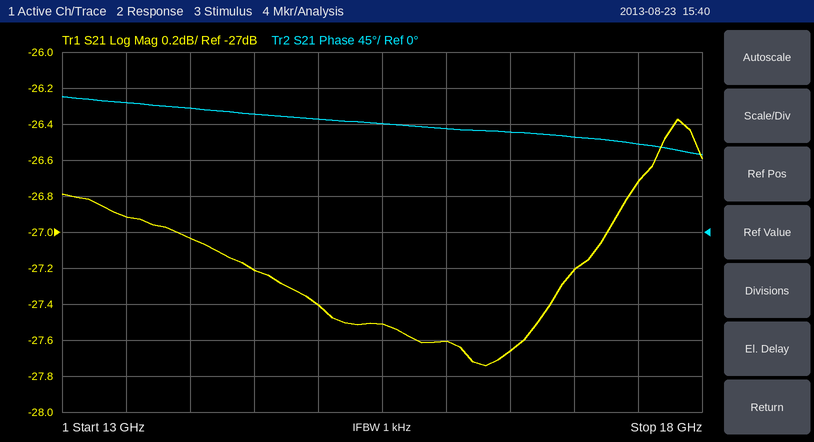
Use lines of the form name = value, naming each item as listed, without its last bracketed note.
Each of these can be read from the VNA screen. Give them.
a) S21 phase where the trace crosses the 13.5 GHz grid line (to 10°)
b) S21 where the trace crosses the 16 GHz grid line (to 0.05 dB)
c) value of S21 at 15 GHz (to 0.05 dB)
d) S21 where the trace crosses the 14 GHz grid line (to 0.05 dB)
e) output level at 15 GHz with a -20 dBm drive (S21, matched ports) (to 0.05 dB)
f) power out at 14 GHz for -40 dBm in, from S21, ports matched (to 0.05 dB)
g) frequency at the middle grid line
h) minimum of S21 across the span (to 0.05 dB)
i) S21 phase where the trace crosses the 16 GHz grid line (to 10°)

S21 phase where the trace crosses the 13.5 GHz grid line = 160°
S21 where the trace crosses the 16 GHz grid line = -27.60 dB
value of S21 at 15 GHz = -27.40 dB
S21 where the trace crosses the 14 GHz grid line = -27.05 dB
output level at 15 GHz with a -20 dBm drive (S21, matched ports) = -47.40 dBm
power out at 14 GHz for -40 dBm in, from S21, ports matched = -67.05 dBm
frequency at the middle grid line = 15.5 GHz
minimum of S21 across the span = -27.75 dB
S21 phase where the trace crosses the 16 GHz grid line = 130°
